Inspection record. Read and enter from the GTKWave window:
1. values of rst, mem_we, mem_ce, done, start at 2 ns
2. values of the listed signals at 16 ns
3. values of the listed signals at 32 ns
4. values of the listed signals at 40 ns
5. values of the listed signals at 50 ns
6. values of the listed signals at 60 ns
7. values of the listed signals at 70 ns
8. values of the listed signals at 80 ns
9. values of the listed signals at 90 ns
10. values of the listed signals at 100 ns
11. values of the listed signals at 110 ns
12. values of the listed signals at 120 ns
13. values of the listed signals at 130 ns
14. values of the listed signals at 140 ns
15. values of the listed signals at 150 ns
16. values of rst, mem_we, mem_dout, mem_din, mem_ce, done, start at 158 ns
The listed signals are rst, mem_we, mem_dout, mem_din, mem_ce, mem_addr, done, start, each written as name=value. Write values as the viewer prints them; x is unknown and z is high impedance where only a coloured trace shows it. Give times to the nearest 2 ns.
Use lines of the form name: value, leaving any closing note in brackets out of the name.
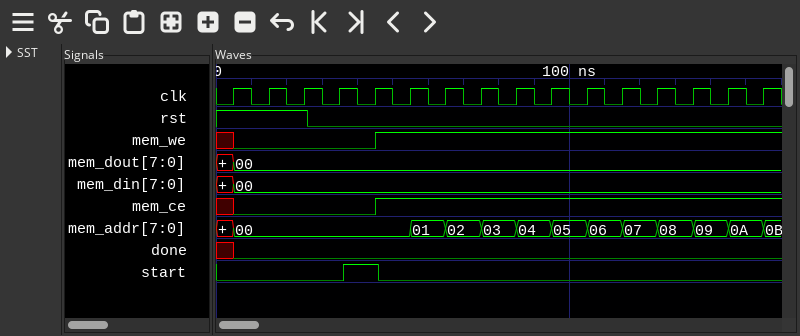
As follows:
values of rst, mem_we, mem_ce, done, start at 2 ns: rst=1, mem_we=x, mem_ce=x, done=x, start=0
values of the listed signals at 16 ns: rst=1, mem_we=0, mem_dout=00, mem_din=00, mem_ce=0, mem_addr=00, done=0, start=0
values of the listed signals at 32 ns: rst=0, mem_we=0, mem_dout=00, mem_din=00, mem_ce=0, mem_addr=00, done=0, start=0
values of the listed signals at 40 ns: rst=0, mem_we=0, mem_dout=00, mem_din=00, mem_ce=0, mem_addr=00, done=0, start=1
values of the listed signals at 50 ns: rst=0, mem_we=1, mem_dout=00, mem_din=00, mem_ce=1, mem_addr=00, done=0, start=0
values of the listed signals at 60 ns: rst=0, mem_we=1, mem_dout=00, mem_din=00, mem_ce=1, mem_addr=01, done=0, start=0
values of the listed signals at 70 ns: rst=0, mem_we=1, mem_dout=00, mem_din=00, mem_ce=1, mem_addr=02, done=0, start=0
values of the listed signals at 80 ns: rst=0, mem_we=1, mem_dout=00, mem_din=00, mem_ce=1, mem_addr=03, done=0, start=0
values of the listed signals at 90 ns: rst=0, mem_we=1, mem_dout=00, mem_din=00, mem_ce=1, mem_addr=04, done=0, start=0
values of the listed signals at 100 ns: rst=0, mem_we=1, mem_dout=00, mem_din=00, mem_ce=1, mem_addr=05, done=0, start=0
values of the listed signals at 110 ns: rst=0, mem_we=1, mem_dout=00, mem_din=00, mem_ce=1, mem_addr=06, done=0, start=0
values of the listed signals at 120 ns: rst=0, mem_we=1, mem_dout=00, mem_din=00, mem_ce=1, mem_addr=07, done=0, start=0
values of the listed signals at 130 ns: rst=0, mem_we=1, mem_dout=00, mem_din=00, mem_ce=1, mem_addr=08, done=0, start=0
values of the listed signals at 140 ns: rst=0, mem_we=1, mem_dout=00, mem_din=00, mem_ce=1, mem_addr=09, done=0, start=0
values of the listed signals at 150 ns: rst=0, mem_we=1, mem_dout=00, mem_din=00, mem_ce=1, mem_addr=0A, done=0, start=0
values of rst, mem_we, mem_dout, mem_din, mem_ce, done, start at 158 ns: rst=0, mem_we=1, mem_dout=00, mem_din=00, mem_ce=1, done=0, start=0
